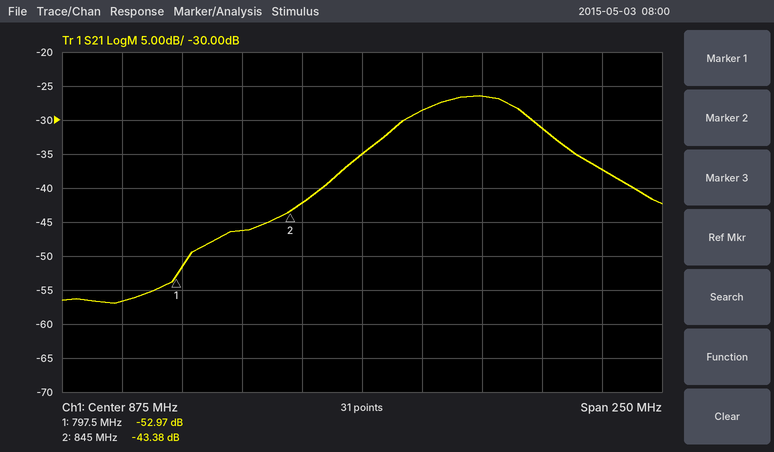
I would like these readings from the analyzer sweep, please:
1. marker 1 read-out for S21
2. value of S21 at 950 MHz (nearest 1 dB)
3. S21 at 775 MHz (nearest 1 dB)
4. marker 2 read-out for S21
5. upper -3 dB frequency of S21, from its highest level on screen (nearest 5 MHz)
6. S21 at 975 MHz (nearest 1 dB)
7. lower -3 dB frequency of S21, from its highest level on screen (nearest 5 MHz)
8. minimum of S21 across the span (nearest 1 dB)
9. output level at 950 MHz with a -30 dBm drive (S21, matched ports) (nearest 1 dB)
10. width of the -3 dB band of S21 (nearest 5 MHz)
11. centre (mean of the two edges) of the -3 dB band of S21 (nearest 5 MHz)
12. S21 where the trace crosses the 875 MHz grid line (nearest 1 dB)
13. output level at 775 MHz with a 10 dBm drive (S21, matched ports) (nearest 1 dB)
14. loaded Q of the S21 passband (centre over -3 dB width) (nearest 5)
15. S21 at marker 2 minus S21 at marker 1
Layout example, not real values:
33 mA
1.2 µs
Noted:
-52.97 dB
-31 dB
-57 dB
-43.38 dB
945 MHz
-37 dB
895 MHz
-57 dB
-61 dBm
50 MHz
920 MHz
-35 dB
-47 dBm
20
9.59 dB
